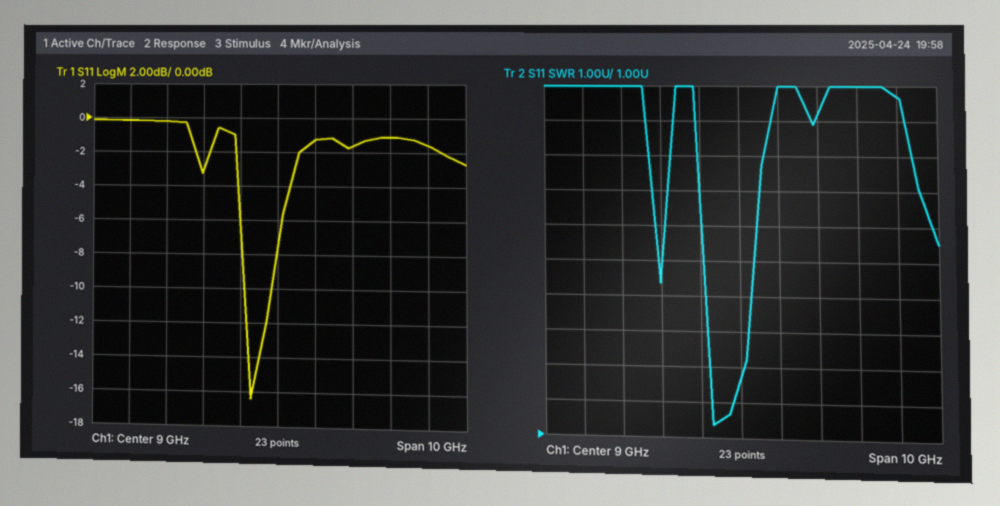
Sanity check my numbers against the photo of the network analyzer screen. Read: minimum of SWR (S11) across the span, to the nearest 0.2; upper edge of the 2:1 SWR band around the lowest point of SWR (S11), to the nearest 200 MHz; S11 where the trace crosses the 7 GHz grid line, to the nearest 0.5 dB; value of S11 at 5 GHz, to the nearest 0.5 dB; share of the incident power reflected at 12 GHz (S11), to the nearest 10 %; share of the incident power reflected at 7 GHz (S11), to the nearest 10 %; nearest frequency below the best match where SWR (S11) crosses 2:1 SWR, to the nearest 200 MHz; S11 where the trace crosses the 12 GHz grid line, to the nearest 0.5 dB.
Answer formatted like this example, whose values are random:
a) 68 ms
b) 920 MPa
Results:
a) 1.4
b) 8.8 GHz
c) -3.0 dB
d) 0.0 dB
e) 80 %
f) 50 %
g) 8.2 GHz
h) -1.0 dB
